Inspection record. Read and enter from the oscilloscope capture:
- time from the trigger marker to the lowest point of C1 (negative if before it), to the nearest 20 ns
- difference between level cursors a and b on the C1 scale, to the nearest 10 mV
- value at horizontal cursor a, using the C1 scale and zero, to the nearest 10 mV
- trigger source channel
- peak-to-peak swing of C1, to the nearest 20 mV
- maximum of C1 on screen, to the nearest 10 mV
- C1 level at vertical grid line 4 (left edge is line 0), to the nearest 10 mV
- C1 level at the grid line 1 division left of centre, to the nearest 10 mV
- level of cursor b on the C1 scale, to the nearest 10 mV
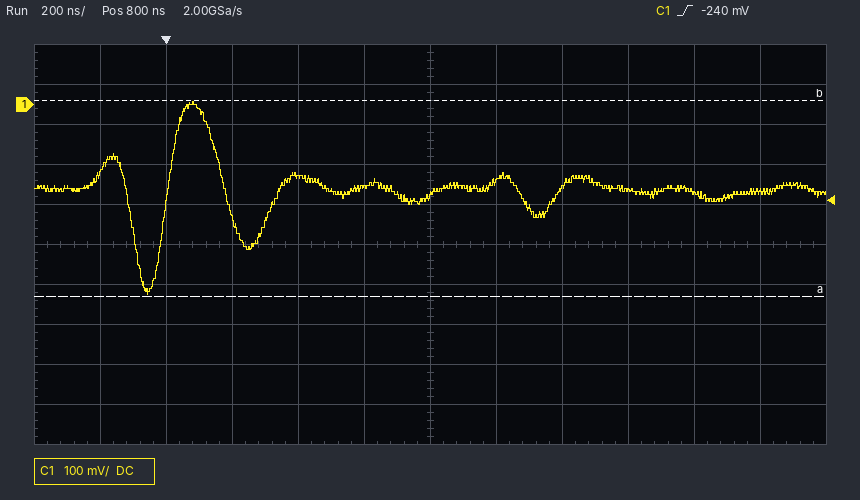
-60 ns
490 mV
-480 mV
C1
480 mV
10 mV
-180 mV
-210 mV
10 mV
